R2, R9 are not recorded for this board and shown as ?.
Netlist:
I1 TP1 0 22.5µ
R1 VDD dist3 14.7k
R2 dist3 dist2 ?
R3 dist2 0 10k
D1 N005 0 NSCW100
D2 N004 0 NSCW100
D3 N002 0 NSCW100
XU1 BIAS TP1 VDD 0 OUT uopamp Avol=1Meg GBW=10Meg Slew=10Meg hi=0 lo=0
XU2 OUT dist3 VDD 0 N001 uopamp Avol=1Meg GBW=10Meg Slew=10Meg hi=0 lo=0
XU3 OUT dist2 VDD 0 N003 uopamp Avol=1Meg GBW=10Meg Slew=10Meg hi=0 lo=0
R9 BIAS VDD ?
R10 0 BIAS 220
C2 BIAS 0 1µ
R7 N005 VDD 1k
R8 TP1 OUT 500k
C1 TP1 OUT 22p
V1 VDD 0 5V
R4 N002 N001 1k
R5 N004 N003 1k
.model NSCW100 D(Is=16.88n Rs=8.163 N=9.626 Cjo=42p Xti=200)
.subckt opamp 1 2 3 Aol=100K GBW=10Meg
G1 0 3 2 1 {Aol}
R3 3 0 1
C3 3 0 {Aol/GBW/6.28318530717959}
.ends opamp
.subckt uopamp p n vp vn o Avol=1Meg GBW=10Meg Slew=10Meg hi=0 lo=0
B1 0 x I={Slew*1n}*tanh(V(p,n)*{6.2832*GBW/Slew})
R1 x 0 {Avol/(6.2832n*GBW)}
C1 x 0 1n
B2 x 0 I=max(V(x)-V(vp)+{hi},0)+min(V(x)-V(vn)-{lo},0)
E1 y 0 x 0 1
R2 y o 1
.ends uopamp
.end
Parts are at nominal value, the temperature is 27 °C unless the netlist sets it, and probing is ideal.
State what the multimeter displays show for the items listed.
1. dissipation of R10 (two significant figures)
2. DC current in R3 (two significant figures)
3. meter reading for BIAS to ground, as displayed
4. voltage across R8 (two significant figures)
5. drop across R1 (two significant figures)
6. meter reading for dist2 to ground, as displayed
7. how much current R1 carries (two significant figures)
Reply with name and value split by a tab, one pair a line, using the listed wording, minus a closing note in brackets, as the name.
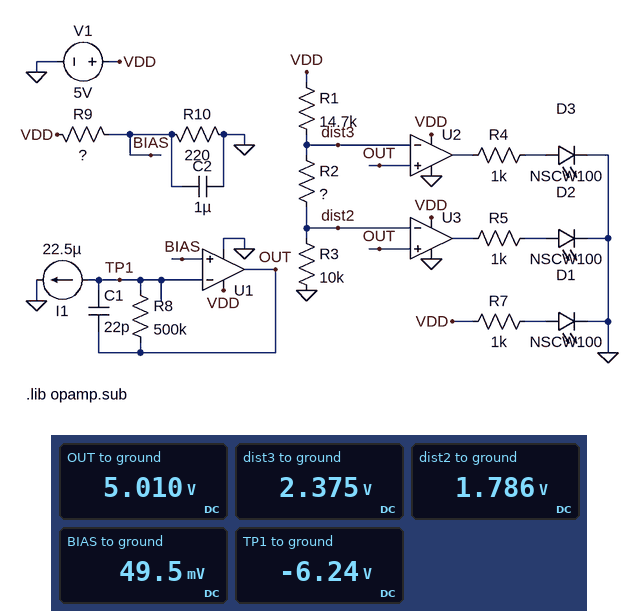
dissipation of R10	11 µW
DC current in R3	180 µA
meter reading for BIAS to ground, as displayed	49.5 mV
voltage across R8	11 V
drop across R1	2.6 V
meter reading for dist2 to ground, as displayed	1.786 V
how much current R1 carries	180 µA
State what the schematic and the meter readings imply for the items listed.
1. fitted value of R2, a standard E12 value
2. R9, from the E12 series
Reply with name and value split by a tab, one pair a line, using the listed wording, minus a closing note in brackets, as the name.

fitted value of R2, a standard E12 value	3.3 kΩ
R9, from the E12 series	22 kΩ
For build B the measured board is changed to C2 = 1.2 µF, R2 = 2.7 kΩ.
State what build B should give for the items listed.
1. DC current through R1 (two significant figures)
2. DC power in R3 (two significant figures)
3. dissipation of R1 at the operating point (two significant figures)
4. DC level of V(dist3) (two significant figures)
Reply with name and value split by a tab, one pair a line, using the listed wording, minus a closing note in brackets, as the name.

DC current through R1	180 µA
DC power in R3	330 µW
dissipation of R1 at the operating point	490 µW
DC level of V(dist3)	2.3 V
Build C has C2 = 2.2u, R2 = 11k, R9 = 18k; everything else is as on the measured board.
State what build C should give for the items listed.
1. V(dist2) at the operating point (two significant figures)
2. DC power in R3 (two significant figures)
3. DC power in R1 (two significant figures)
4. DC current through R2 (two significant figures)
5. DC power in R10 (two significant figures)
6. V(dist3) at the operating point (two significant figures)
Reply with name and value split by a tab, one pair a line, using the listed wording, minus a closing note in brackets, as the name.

V(dist2) at the operating point	1.4 V
DC power in R3	200 µW
DC power in R1	290 µW
DC current through R2	140 µA
DC power in R10	17 µW
V(dist3) at the operating point	2.9 V
